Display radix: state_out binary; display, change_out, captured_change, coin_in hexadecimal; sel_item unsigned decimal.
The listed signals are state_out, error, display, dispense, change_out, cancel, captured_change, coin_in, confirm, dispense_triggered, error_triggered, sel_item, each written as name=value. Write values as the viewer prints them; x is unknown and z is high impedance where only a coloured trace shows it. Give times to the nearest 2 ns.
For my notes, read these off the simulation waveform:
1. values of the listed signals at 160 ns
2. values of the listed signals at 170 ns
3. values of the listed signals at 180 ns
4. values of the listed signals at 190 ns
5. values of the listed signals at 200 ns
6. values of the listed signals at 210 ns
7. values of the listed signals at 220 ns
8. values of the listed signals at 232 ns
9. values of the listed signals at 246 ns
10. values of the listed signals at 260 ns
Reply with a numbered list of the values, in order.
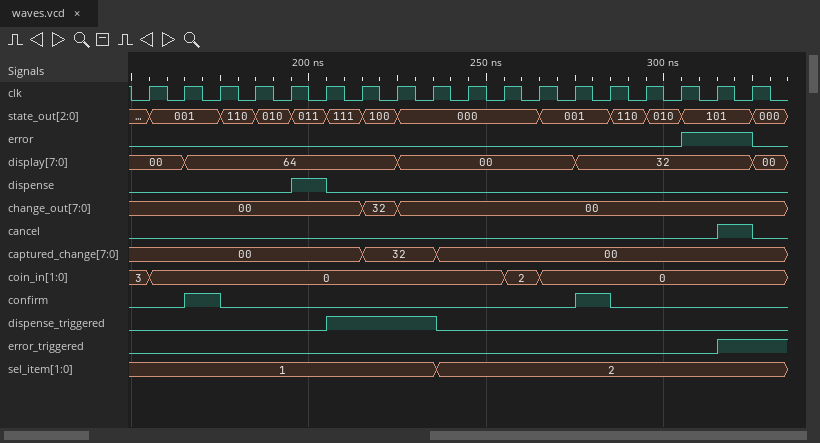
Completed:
1. state_out=001, error=0, display=00, dispense=0, change_out=00, cancel=0, captured_change=00, coin_in=0, confirm=0, dispense_triggered=0, error_triggered=0, sel_item=1
2. state_out=001, error=0, display=64, dispense=0, change_out=00, cancel=0, captured_change=00, coin_in=0, confirm=1, dispense_triggered=0, error_triggered=0, sel_item=1
3. state_out=110, error=0, display=64, dispense=0, change_out=00, cancel=0, captured_change=00, coin_in=0, confirm=0, dispense_triggered=0, error_triggered=0, sel_item=1
4. state_out=010, error=0, display=64, dispense=0, change_out=00, cancel=0, captured_change=00, coin_in=0, confirm=0, dispense_triggered=0, error_triggered=0, sel_item=1
5. state_out=011, error=0, display=64, dispense=1, change_out=00, cancel=0, captured_change=00, coin_in=0, confirm=0, dispense_triggered=0, error_triggered=0, sel_item=1
6. state_out=111, error=0, display=64, dispense=0, change_out=00, cancel=0, captured_change=00, coin_in=0, confirm=0, dispense_triggered=1, error_triggered=0, sel_item=1
7. state_out=100, error=0, display=64, dispense=0, change_out=32, cancel=0, captured_change=32, coin_in=0, confirm=0, dispense_triggered=1, error_triggered=0, sel_item=1
8. state_out=000, error=0, display=00, dispense=0, change_out=00, cancel=0, captured_change=32, coin_in=0, confirm=0, dispense_triggered=1, error_triggered=0, sel_item=1
9. state_out=000, error=0, display=00, dispense=0, change_out=00, cancel=0, captured_change=00, coin_in=0, confirm=0, dispense_triggered=0, error_triggered=0, sel_item=2
10. state_out=000, error=0, display=00, dispense=0, change_out=00, cancel=0, captured_change=00, coin_in=2, confirm=0, dispense_triggered=0, error_triggered=0, sel_item=2
